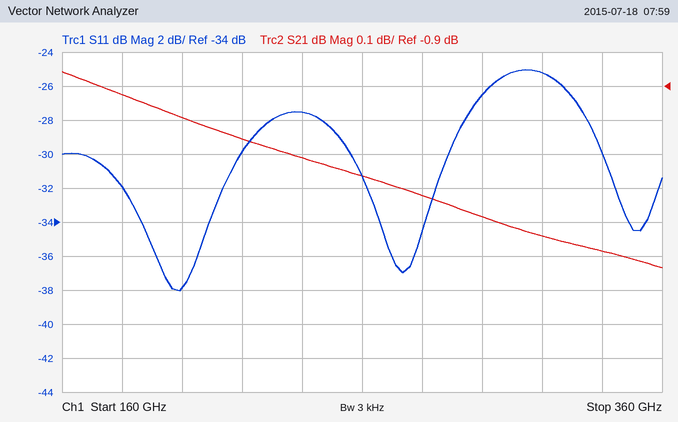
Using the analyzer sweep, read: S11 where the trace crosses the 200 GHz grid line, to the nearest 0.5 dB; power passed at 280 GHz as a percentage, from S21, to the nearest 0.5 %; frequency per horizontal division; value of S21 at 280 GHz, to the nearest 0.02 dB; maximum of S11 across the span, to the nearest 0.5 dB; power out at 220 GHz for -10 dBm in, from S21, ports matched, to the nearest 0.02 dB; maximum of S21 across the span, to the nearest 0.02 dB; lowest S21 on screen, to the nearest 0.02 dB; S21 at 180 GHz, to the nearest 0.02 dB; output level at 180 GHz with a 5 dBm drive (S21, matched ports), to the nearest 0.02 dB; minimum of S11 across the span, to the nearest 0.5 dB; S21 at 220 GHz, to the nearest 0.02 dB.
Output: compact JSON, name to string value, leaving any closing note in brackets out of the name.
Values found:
{"S11 where the trace crosses the 200 GHz grid line, to the nearest 0.5 dB": "-38.0 dB", "power passed at 280 GHz as a percentage, from S21, to the nearest 0.5 %": "75.5 %", "frequency per horizontal division": "20 GHz", "value of S21 at 280 GHz, to the nearest 0.02 dB": "-1.22 dB", "maximum of S11 across the span, to the nearest 0.5 dB": "-25.0 dB", "power out at 220 GHz for -10 dBm in, from S21, ports matched, to the nearest 0.02 dB": "-11.06 dBm", "maximum of S21 across the span, to the nearest 0.02 dB": "-0.86 dB", "lowest S21 on screen, to the nearest 0.02 dB": "-1.44 dB", "S21 at 180 GHz, to the nearest 0.02 dB": "-0.92 dB", "output level at 180 GHz with a 5 dBm drive (S21, matched ports), to the nearest 0.02 dB": "4.08 dBm", "minimum of S11 across the span, to the nearest 0.5 dB": "-38.0 dB", "S21 at 220 GHz, to the nearest 0.02 dB": "-1.06 dB"}
